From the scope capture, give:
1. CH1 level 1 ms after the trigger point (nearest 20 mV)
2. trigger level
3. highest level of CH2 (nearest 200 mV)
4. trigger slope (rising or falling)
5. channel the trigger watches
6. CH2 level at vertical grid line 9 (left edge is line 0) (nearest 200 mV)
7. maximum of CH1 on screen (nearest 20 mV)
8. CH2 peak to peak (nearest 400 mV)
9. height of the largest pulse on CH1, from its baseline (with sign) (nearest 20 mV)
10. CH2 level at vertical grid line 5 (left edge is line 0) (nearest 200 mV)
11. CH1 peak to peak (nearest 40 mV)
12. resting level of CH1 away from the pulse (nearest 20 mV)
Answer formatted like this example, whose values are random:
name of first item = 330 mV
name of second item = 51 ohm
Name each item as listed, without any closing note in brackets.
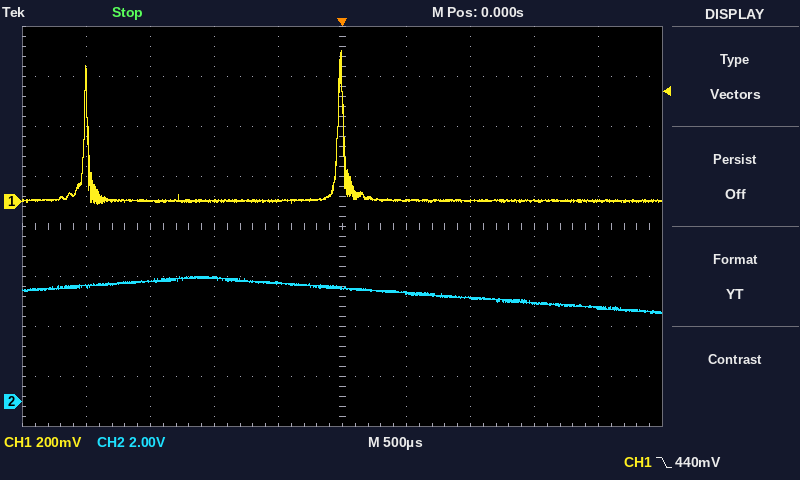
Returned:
CH1 level 1 ms after the trigger point = 0 mV
trigger level = 440 mV
highest level of CH2 = 5.0 V
trigger slope = falling
channel the trigger watches = CH1
CH2 level at vertical grid line 9 (left edge is line 0) = 3.8 V
maximum of CH1 on screen = 600 mV
CH2 peak to peak = 1.6 V
height of the largest pulse on CH1, from its baseline (with sign) = +600 mV
CH2 level at vertical grid line 5 (left edge is line 0) = 4.6 V
CH1 peak to peak = 600 mV
resting level of CH1 away from the pulse = 0 mV
